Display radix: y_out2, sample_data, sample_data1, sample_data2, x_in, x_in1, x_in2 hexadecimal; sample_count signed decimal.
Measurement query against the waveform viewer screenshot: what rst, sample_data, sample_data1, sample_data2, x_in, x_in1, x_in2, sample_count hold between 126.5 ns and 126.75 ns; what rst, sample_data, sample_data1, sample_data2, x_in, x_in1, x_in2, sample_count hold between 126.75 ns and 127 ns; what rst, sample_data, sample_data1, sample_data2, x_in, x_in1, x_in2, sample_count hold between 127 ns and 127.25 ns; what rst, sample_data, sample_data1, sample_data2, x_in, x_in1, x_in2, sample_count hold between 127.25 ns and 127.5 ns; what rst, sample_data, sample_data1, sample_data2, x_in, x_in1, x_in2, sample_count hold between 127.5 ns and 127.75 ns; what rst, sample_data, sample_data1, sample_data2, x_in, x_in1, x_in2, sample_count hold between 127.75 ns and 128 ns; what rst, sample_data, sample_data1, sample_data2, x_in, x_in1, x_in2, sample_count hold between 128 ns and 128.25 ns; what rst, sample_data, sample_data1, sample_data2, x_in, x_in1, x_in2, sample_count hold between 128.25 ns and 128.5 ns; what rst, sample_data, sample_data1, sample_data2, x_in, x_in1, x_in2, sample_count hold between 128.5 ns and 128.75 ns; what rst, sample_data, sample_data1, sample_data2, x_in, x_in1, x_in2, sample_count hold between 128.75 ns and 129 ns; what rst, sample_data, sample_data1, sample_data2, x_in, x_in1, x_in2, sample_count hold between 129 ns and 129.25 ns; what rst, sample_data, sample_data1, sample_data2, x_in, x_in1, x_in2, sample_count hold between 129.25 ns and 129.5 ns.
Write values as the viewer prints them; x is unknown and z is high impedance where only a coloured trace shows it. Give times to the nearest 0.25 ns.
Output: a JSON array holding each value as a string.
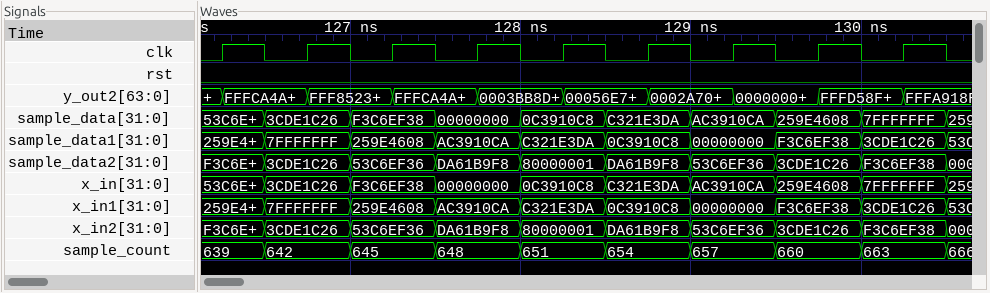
["rst=0, sample_data=3CDE1C26, sample_data1=7FFFFFFF, sample_data2=3CDE1C26, x_in=3CDE1C26, x_in1=7FFFFFFF, x_in2=3CDE1C26, sample_count=642", "rst=0, sample_data=3CDE1C26, sample_data1=7FFFFFFF, sample_data2=3CDE1C26, x_in=3CDE1C26, x_in1=7FFFFFFF, x_in2=3CDE1C26, sample_count=642", "rst=0, sample_data=F3C6EF38, sample_data1=259E4608, sample_data2=53C6EF36, x_in=F3C6EF38, x_in1=259E4608, x_in2=53C6EF36, sample_count=645", "rst=0, sample_data=F3C6EF38, sample_data1=259E4608, sample_data2=53C6EF36, x_in=F3C6EF38, x_in1=259E4608, x_in2=53C6EF36, sample_count=645", "rst=0, sample_data=00000000, sample_data1=AC3910CA, sample_data2=DA61B9F8, x_in=00000000, x_in1=AC3910CA, x_in2=DA61B9F8, sample_count=648", "rst=0, sample_data=00000000, sample_data1=AC3910CA, sample_data2=DA61B9F8, x_in=00000000, x_in1=AC3910CA, x_in2=DA61B9F8, sample_count=648", "rst=0, sample_data=0C3910C8, sample_data1=C321E3DA, sample_data2=80000001, x_in=0C3910C8, x_in1=C321E3DA, x_in2=80000001, sample_count=651", "rst=0, sample_data=0C3910C8, sample_data1=C321E3DA, sample_data2=80000001, x_in=0C3910C8, x_in1=C321E3DA, x_in2=80000001, sample_count=651", "rst=0, sample_data=C321E3DA, sample_data1=0C3910C8, sample_data2=DA61B9F8, x_in=C321E3DA, x_in1=0C3910C8, x_in2=DA61B9F8, sample_count=654", "rst=0, sample_data=C321E3DA, sample_data1=0C3910C8, sample_data2=DA61B9F8, x_in=C321E3DA, x_in1=0C3910C8, x_in2=DA61B9F8, sample_count=654", "rst=0, sample_data=AC3910CA, sample_data1=00000000, sample_data2=53C6EF36, x_in=AC3910CA, x_in1=00000000, x_in2=53C6EF36, sample_count=657", "rst=0, sample_data=AC3910CA, sample_data1=00000000, sample_data2=53C6EF36, x_in=AC3910CA, x_in1=00000000, x_in2=53C6EF36, sample_count=657"]
